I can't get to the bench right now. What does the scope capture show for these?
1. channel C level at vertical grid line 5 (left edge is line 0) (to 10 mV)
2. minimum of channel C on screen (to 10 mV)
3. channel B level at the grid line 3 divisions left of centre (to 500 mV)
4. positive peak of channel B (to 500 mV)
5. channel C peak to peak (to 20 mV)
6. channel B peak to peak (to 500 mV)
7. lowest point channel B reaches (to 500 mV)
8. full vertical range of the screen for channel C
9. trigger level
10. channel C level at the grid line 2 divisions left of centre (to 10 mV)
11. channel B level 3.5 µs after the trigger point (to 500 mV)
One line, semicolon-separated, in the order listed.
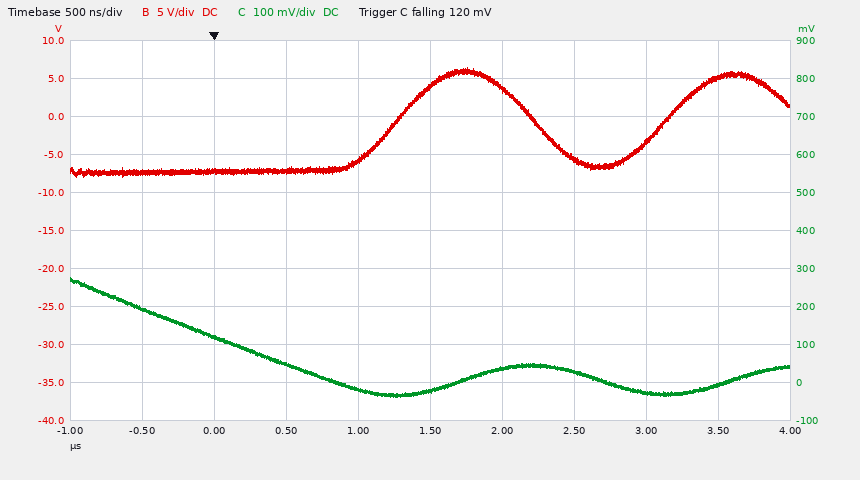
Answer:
-20 mV; -40 mV; -7.0 V; 6.5 V; 320 mV; 14.5 V; -8.0 V; 1 V; 120 mV; 50 mV; 5.0 V
